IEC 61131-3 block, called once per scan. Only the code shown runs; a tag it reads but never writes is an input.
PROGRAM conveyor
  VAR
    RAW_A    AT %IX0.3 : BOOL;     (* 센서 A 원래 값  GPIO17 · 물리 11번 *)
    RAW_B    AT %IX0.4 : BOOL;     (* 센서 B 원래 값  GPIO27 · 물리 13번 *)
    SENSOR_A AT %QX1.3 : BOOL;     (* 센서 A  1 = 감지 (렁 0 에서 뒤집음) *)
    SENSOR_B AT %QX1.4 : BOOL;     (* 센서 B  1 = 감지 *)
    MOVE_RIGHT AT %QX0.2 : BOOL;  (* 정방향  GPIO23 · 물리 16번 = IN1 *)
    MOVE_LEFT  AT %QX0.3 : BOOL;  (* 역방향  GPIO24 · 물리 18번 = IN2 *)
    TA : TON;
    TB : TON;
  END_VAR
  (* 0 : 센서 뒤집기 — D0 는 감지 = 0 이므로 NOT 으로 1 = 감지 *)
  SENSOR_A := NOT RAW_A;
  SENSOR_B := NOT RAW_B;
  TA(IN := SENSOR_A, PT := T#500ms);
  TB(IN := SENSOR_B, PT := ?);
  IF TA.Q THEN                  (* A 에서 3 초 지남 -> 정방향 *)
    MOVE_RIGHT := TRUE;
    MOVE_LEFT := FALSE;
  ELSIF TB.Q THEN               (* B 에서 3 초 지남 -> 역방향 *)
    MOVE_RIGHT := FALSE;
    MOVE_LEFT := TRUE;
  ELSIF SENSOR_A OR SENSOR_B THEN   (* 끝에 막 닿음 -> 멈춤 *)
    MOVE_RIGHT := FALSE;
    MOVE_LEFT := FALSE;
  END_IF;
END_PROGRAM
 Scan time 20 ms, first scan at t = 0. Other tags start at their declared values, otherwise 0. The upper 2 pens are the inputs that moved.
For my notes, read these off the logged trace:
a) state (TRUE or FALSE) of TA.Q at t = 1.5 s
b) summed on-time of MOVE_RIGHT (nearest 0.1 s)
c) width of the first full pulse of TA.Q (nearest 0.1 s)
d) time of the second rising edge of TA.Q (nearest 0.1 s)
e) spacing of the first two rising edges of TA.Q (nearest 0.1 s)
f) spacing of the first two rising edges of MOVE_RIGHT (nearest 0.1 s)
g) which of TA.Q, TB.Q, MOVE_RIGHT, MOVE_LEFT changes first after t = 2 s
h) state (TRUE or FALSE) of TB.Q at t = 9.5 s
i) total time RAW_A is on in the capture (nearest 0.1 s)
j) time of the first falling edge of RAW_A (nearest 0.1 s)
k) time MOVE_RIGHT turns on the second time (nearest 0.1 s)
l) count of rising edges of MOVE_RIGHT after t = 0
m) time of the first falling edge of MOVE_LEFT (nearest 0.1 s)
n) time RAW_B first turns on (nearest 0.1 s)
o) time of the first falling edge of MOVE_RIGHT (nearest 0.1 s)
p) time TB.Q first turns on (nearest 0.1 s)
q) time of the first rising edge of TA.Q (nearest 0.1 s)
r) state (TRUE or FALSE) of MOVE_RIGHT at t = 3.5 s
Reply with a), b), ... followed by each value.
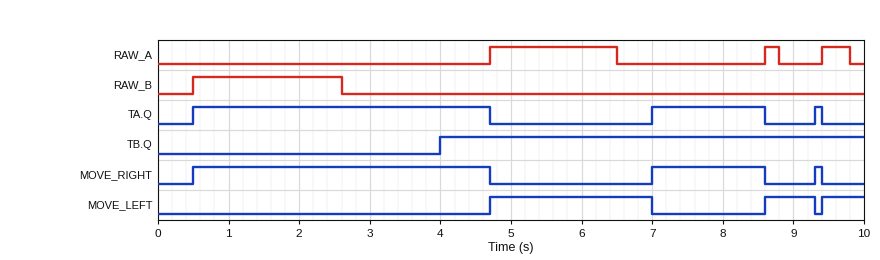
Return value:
a) TRUE
b) 5.9 s
c) 4.2 s
d) 7.0 s
e) 6.5 s
f) 6.5 s
g) TB.Q
h) TRUE
i) 2.4 s
j) 6.5 s
k) 7.0 s
l) 3
m) 7.0 s
n) 0.5 s
o) 4.7 s
p) 4.0 s
q) 0.5 s
r) TRUE
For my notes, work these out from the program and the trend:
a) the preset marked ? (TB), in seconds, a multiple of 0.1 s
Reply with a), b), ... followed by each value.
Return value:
a) 1.4 s
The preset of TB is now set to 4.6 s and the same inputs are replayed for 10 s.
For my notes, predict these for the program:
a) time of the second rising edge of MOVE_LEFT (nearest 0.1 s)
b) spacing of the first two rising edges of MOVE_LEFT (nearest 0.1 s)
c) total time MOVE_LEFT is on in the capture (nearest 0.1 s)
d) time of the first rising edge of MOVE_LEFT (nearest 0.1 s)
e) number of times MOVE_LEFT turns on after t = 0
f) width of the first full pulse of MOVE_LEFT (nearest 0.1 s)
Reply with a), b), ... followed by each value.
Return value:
a) 9.4 s
b) 0.8 s
c) 1.3 s
d) 8.6 s
e) 2
f) 0.7 s
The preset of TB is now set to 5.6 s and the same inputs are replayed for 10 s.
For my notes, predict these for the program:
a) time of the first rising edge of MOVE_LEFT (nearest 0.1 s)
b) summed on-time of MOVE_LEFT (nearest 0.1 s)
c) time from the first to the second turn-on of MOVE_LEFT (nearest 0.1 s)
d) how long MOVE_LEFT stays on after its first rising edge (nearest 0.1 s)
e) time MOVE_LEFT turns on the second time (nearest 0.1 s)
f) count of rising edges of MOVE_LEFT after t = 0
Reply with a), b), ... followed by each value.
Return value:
a) 8.6 s
b) 1.3 s
c) 0.8 s
d) 0.7 s
e) 9.4 s
f) 2
